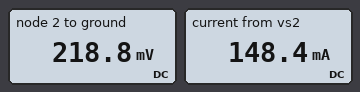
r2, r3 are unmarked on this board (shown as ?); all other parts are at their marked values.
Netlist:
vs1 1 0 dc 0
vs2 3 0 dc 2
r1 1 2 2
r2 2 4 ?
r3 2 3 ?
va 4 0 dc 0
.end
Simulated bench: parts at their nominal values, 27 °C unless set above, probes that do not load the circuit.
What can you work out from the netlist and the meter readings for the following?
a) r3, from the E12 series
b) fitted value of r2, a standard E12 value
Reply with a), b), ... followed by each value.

a) 12 Ω
b) 5.6 Ω
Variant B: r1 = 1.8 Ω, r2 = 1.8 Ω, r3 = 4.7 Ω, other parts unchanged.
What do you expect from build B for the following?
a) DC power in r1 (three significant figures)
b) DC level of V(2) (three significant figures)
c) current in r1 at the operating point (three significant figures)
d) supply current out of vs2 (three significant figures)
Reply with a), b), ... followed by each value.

a) 57.4 mW
b) 321 mV
c) 179 mA
d) 357 mA
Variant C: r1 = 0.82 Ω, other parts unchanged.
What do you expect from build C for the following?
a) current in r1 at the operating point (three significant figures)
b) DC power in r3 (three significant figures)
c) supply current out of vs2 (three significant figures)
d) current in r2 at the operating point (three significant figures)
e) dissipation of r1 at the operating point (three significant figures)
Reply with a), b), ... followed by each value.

a) 137 mA
b) 297 mW
c) 157 mA
d) 20.1 mA
e) 15.4 mW
